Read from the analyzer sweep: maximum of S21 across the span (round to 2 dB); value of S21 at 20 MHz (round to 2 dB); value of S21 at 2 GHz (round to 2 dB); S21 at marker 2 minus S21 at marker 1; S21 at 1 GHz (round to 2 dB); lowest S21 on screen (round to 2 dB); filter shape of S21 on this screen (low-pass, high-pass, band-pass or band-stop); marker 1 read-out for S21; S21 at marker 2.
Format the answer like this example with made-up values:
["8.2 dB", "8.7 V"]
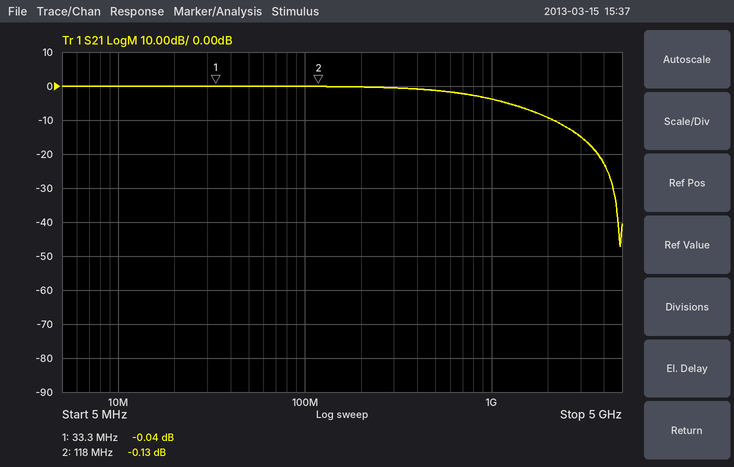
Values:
["0 dB", "0 dB", "-10 dB", "-0.09 dB", "-4 dB", "-48 dB", "low-pass", "-0.04 dB", "-0.13 dB"]
